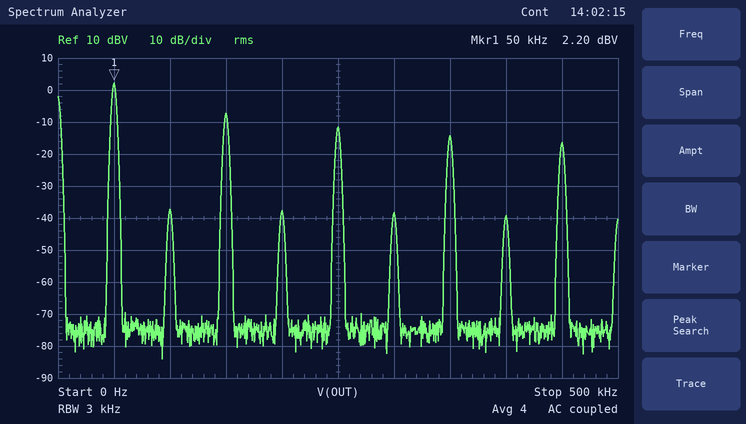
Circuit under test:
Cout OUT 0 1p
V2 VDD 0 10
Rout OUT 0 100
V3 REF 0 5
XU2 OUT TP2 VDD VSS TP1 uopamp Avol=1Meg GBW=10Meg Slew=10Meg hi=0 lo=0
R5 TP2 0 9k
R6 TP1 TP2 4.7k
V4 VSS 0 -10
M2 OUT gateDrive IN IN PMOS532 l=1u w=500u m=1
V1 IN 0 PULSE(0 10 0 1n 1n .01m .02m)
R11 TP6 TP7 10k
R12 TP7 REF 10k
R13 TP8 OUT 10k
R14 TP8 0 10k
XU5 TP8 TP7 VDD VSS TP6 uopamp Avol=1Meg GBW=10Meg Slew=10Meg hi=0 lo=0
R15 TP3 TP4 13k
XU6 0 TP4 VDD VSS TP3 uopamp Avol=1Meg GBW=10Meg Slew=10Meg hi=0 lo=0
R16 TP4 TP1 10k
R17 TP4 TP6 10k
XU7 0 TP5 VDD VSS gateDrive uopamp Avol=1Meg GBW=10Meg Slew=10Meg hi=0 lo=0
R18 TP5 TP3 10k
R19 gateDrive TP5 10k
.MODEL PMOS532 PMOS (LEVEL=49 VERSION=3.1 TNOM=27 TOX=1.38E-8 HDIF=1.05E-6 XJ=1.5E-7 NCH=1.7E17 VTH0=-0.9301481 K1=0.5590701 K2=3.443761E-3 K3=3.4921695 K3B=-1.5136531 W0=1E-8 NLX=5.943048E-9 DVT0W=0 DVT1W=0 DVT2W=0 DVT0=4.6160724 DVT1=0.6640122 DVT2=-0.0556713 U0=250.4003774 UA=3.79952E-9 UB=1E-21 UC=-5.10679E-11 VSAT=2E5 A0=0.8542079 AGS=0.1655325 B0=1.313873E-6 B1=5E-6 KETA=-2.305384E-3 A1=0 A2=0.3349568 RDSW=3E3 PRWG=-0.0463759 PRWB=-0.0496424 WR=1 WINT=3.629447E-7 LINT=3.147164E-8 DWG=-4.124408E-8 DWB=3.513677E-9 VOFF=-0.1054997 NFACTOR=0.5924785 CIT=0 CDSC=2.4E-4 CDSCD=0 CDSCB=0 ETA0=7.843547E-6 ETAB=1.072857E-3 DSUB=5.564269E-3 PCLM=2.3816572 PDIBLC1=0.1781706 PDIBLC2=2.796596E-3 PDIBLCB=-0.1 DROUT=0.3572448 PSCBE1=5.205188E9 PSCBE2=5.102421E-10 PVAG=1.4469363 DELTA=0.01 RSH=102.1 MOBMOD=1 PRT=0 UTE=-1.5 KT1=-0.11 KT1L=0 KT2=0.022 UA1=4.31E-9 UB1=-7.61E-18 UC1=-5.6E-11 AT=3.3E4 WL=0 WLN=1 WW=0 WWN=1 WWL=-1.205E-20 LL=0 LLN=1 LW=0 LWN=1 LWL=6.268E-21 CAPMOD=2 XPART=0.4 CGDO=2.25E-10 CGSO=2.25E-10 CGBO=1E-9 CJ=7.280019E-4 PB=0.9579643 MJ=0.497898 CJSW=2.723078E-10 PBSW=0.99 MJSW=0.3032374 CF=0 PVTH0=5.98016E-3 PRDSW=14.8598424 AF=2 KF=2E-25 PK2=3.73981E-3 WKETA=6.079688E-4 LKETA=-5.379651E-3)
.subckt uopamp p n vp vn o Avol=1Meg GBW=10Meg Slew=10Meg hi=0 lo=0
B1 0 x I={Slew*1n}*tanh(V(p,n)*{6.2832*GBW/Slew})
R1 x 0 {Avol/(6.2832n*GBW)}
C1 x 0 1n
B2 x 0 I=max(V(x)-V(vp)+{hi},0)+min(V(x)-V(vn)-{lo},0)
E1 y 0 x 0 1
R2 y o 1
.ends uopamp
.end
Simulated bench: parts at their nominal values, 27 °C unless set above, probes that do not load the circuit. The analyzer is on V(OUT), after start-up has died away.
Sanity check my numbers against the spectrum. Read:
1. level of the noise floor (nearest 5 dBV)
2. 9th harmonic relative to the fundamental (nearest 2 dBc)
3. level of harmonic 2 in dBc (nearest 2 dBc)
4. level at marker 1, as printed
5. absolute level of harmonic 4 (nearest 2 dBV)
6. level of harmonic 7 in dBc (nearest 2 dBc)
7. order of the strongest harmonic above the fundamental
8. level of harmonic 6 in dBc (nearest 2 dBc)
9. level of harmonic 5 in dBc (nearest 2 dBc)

-75 dBV
-18 dBc
-40 dBc
2.20 dBV
-38 dBV
-16 dBc
3
-40 dBc
-14 dBc
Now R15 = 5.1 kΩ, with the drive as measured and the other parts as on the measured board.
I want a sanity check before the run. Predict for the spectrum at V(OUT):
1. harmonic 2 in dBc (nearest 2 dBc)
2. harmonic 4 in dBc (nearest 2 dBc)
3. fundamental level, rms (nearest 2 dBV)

-56 dBc
-56 dBc
2 dBV
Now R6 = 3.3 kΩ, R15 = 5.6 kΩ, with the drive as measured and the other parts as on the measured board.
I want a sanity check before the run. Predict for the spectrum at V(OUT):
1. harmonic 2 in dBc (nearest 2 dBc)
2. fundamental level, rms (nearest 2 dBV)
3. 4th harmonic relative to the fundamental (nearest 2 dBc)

-56 dBc
2 dBV
-56 dBc
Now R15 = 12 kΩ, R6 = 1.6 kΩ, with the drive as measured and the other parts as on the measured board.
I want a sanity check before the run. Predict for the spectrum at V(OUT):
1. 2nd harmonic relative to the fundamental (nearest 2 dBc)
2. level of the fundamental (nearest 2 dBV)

-46 dBc
2 dBV
